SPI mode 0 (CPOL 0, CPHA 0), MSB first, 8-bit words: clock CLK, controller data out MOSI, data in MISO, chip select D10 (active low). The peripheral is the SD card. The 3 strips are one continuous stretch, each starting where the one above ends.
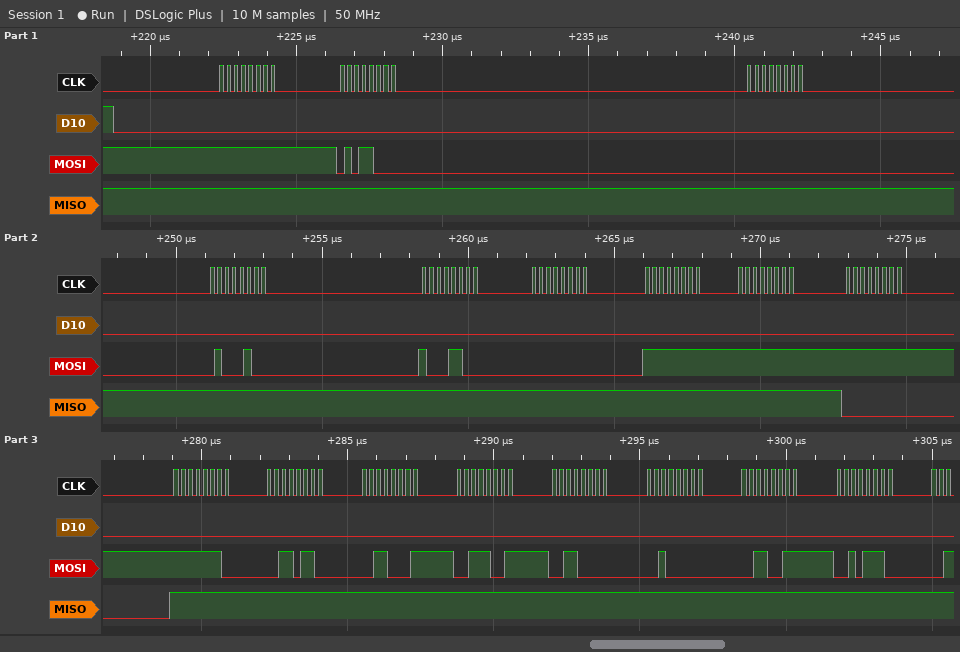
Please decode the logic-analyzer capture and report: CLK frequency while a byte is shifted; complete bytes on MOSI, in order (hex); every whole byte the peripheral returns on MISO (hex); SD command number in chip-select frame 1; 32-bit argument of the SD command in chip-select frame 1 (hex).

4 MHz
FF 58 00 44 8C 00 FF FF FF FE 36 31 39 30 20 33 2E
FF FF FF FF FF FF FF FF 00 FF FF FF FF FF FF FF FF
CMD24
0x00448C00
